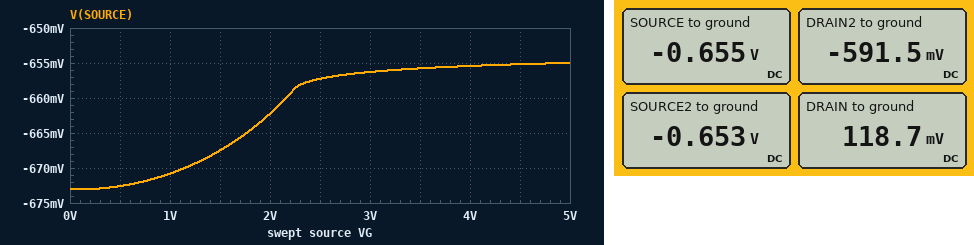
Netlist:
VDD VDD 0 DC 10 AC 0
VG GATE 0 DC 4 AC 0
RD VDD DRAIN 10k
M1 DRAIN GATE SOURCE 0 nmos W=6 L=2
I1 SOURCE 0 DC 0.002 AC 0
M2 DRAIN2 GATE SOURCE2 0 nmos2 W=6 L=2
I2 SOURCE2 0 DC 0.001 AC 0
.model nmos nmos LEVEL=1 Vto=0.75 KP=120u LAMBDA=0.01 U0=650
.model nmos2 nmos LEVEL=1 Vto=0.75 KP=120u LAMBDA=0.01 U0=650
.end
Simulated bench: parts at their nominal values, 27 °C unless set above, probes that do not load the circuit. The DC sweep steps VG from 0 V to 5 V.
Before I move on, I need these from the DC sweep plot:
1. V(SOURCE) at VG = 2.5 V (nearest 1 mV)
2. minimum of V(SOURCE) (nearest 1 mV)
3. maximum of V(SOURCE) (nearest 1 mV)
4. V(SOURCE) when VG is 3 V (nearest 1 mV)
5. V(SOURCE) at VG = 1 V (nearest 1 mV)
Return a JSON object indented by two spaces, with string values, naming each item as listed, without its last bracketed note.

{
  "V(SOURCE) at VG = 2.5 V": "-657 mV",
  "minimum of V(SOURCE)": "-673 mV",
  "maximum of V(SOURCE)": "-655 mV",
  "V(SOURCE) when VG is 3 V": "-656 mV",
  "V(SOURCE) at VG = 1 V": "-671 mV"
}
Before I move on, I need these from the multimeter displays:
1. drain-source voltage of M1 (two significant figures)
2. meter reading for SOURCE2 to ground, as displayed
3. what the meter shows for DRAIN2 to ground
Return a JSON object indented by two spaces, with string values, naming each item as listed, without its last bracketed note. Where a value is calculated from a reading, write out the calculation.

{
  "drain-source voltage of M1": "118.7 mV - (-655 mV) = 770 mV",
  "meter reading for SOURCE2 to ground, as displayed": "-0.653 V",
  "what the meter shows for DRAIN2 to ground": "-591.5 mV"
}
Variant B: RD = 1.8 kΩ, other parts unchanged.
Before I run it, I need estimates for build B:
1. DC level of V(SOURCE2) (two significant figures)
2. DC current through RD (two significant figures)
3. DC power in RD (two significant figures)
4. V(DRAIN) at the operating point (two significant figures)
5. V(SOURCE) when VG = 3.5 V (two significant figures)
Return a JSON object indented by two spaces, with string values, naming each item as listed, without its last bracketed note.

{
  "DC level of V(SOURCE2)": "-650 mV",
  "DC current through RD": "2.0 mA",
  "DC power in RD": "7.2 mW",
  "V(DRAIN) at the operating point": "6.4 V",
  "V(SOURCE) when VG = 3.5 V": "-470 mV"
}
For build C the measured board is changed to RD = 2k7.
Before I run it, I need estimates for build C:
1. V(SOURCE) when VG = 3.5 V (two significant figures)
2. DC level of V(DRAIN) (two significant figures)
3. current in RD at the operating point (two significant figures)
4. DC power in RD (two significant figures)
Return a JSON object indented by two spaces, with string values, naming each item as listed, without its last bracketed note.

{
  "V(SOURCE) when VG = 3.5 V": "-500 mV",
  "DC level of V(DRAIN)": "4.6 V",
  "current in RD at the operating point": "2.0 mA",
  "DC power in RD": "11 mW"
}
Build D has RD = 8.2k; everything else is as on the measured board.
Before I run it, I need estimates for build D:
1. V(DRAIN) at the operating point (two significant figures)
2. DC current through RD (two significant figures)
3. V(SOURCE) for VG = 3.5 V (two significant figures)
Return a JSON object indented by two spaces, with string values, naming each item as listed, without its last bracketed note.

{
  "V(DRAIN) at the operating point": "300 mV",
  "DC current through RD": "1.2 mA",
  "V(SOURCE) for VG = 3.5 V": "-650 mV"
}
